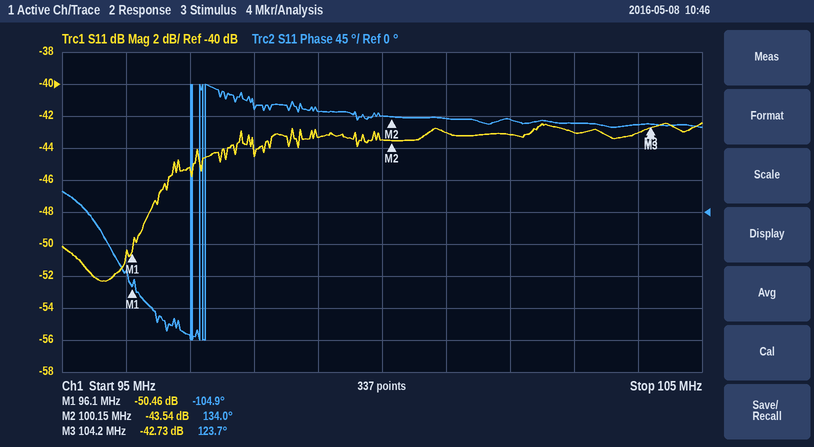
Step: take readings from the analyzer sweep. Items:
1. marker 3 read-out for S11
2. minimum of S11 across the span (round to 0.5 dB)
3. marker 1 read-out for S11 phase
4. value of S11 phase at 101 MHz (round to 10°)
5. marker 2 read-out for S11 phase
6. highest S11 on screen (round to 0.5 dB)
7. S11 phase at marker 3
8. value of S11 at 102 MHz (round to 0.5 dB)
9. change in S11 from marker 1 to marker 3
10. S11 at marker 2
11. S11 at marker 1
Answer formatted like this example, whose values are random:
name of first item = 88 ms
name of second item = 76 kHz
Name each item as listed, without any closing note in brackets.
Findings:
marker 3 read-out for S11 = -42.73 dB
minimum of S11 across the span = -52.5 dB
marker 1 read-out for S11 phase = -104.9°
value of S11 phase at 101 MHz = 130°
marker 2 read-out for S11 phase = 134.0°
highest S11 on screen = -42.5 dB
S11 phase at marker 3 = 123.7°
value of S11 at 102 MHz = -43.0 dB
change in S11 from marker 1 to marker 3 = 7.73 dB
S11 at marker 2 = -43.54 dB
S11 at marker 1 = -50.46 dB
